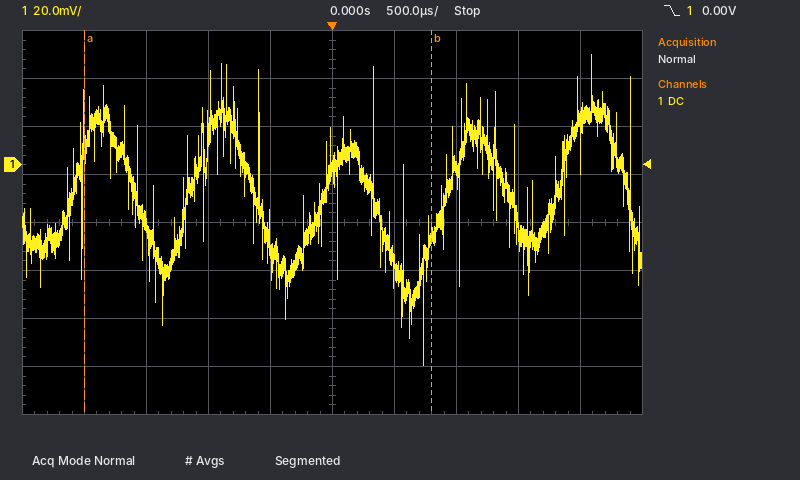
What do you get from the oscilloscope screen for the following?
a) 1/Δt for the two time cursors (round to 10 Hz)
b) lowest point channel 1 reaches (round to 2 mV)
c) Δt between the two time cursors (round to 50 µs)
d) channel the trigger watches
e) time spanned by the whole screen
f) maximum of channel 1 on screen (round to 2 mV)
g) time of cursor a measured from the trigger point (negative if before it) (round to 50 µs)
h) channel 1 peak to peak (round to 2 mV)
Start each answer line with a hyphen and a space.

- 360 Hz
- -84 mV
- 2.80 ms
- channel 1
- 5 ms
- 46 mV
- -2.00 ms
- 130 mV
